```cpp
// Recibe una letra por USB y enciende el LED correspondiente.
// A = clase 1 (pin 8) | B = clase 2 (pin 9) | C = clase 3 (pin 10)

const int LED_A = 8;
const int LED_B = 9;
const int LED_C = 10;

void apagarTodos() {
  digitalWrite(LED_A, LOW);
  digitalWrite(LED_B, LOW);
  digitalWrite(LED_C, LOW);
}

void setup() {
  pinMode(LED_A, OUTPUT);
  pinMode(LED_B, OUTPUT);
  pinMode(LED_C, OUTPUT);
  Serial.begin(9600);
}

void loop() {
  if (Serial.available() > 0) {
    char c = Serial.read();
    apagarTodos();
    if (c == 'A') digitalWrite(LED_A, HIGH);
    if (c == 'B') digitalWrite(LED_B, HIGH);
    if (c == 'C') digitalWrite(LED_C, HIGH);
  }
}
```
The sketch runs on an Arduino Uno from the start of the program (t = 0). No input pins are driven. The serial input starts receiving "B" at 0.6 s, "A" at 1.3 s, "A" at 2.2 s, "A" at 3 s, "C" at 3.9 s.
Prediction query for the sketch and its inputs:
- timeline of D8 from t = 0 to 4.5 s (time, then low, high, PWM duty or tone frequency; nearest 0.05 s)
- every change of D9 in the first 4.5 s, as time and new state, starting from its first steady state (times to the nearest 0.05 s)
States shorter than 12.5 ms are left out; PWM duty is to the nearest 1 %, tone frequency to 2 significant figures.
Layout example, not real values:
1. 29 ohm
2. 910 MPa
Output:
1. 0 s low; 1.3 s high; 3.9 s low
2. 0 s low; 0.6 s high; 1.3 s low
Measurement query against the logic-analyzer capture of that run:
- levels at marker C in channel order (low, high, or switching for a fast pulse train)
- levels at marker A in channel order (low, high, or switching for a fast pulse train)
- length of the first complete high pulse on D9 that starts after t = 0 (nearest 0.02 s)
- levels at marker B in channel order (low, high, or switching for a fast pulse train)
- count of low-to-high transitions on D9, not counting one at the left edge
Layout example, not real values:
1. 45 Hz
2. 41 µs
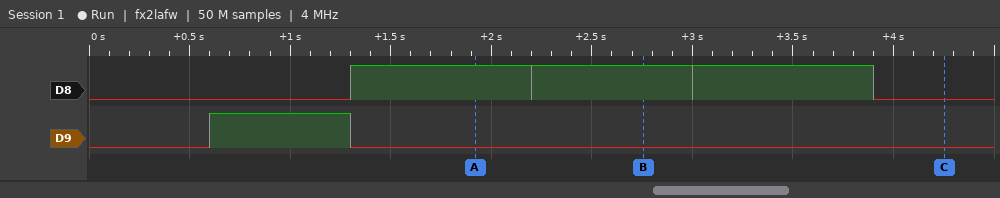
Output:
1. D8 low, D9 low
2. D8 high, D9 low
3. 0.70 s
4. D8 high, D9 low
5. 1
